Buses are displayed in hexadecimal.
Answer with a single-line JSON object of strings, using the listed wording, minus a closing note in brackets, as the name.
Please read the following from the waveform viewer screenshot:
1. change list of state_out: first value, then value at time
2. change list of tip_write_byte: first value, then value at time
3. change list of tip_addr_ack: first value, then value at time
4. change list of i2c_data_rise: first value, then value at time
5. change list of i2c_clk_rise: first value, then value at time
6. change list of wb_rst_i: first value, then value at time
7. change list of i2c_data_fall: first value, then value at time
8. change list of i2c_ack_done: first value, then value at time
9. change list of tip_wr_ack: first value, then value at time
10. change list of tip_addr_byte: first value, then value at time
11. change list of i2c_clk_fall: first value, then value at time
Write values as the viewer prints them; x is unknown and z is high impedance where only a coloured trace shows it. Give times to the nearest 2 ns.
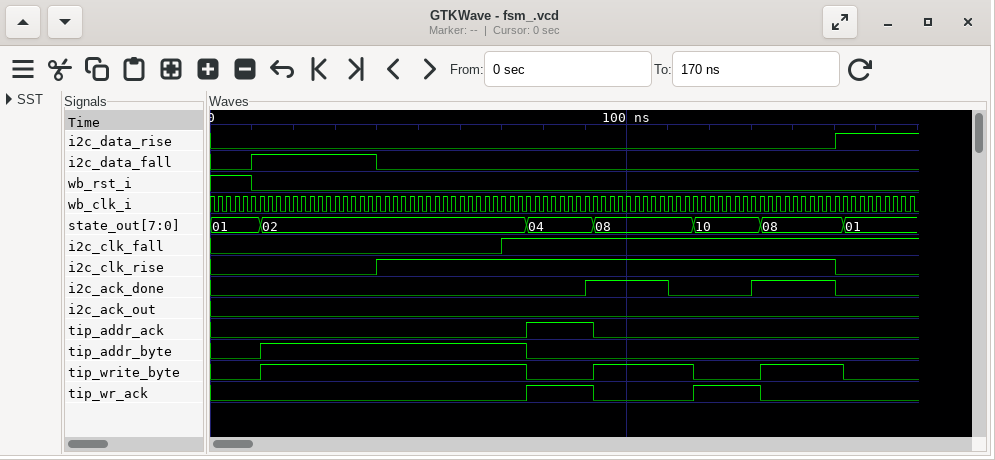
{"change list of state_out: first value, then value at time": "01, 02 at 12 ns, 04 at 76 ns, 08 at 92 ns, 10 at 116 ns, 08 at 132 ns, 01 at 152 ns", "change list of tip_write_byte: first value, then value at time": "0, 1 at 12 ns, 0 at 76 ns, 1 at 92 ns, 0 at 116 ns, 1 at 132 ns, 0 at 152 ns", "change list of tip_addr_ack: first value, then value at time": "0, 1 at 76 ns, 0 at 92 ns", "change list of i2c_data_rise: first value, then value at time": "0, 1 at 150 ns", "change list of i2c_clk_rise: first value, then value at time": "0, 1 at 40 ns, 0 at 150 ns", "change list of wb_rst_i: first value, then value at time": "1, 0 at 10 ns", "change list of i2c_data_fall: first value, then value at time": "0, 1 at 10 ns, 0 at 40 ns", "change list of i2c_ack_done: first value, then value at time": "0, 1 at 90 ns, 0 at 110 ns, 1 at 130 ns, 0 at 150 ns", "change list of tip_wr_ack: first value, then value at time": "0, 1 at 76 ns, 0 at 92 ns, 1 at 116 ns, 0 at 132 ns", "change list of tip_addr_byte: first value, then value at time": "0, 1 at 12 ns, 0 at 76 ns", "change list of i2c_clk_fall: first value, then value at time": "0, 1 at 70 ns"}
